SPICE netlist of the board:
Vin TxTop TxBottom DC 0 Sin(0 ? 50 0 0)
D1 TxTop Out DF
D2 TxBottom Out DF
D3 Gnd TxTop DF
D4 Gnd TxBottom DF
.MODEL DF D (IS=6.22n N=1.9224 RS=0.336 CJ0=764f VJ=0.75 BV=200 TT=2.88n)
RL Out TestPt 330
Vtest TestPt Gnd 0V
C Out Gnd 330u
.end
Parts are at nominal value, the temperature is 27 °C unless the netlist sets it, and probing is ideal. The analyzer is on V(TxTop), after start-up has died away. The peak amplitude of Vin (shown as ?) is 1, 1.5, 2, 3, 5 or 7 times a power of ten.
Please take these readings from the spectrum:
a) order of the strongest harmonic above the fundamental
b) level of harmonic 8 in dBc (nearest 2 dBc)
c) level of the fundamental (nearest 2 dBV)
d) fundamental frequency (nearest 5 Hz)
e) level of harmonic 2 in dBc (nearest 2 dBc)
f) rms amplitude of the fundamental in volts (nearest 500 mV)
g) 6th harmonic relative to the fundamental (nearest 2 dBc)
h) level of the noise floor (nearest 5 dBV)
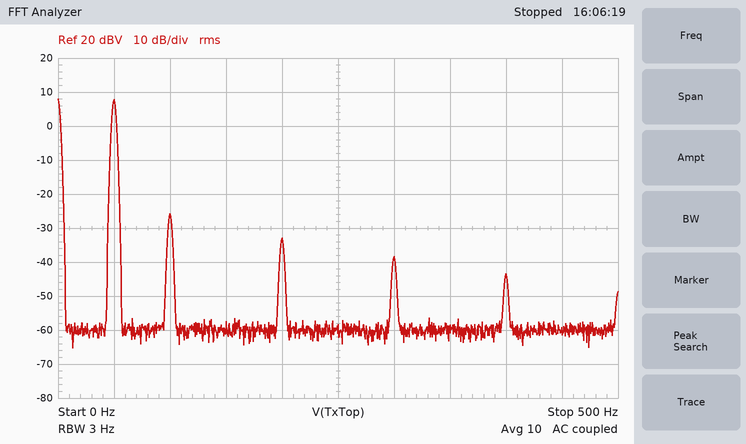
2
-52 dBc
8 dBV
50 Hz
-34 dBc
2.5 V
-46 dBc
-60 dBV
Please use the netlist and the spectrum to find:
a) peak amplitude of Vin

7 V
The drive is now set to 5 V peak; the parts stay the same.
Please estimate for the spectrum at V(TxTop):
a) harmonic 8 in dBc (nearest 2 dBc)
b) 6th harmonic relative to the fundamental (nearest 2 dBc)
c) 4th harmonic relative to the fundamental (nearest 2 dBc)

-54 dBc
-48 dBc
-42 dBc
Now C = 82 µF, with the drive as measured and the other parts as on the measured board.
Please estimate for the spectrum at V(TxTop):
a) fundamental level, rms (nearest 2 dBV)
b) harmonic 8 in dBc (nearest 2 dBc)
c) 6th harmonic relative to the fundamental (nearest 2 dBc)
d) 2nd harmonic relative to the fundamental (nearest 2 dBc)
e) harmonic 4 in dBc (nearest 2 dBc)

8 dBV
-44 dBc
-38 dBc
-22 dBc
-30 dBc
